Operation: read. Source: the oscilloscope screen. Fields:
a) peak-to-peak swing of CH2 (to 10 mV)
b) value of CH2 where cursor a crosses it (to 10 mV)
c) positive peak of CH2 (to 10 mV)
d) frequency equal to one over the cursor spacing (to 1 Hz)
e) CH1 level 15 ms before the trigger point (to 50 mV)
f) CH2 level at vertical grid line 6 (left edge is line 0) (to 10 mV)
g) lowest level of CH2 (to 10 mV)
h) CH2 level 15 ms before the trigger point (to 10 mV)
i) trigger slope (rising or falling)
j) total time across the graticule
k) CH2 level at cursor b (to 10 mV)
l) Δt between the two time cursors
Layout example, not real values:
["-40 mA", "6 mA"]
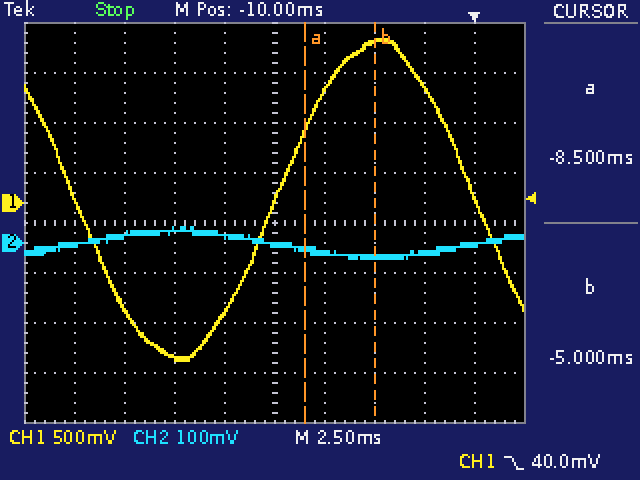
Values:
["60 mV", "-20 mV", "30 mV", "286 Hz", "-1.55 V", "-20 mV", "-30 mV", "30 mV", "falling", "25 ms", "-30 mV", "3.50 ms"]
